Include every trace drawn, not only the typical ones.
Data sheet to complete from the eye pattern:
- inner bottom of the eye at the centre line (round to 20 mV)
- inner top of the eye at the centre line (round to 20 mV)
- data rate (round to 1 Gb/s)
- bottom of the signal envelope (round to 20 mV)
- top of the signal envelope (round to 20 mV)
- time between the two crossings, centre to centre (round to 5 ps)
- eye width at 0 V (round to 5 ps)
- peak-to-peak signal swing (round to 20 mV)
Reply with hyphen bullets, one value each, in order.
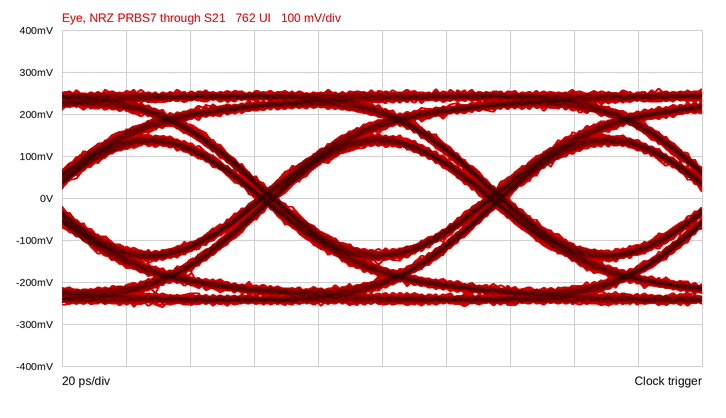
- -120 mV
- 120 mV
- 14 Gb/s
- -260 mV
- 260 mV
- 70 ps
- 65 ps
- 520 mV
